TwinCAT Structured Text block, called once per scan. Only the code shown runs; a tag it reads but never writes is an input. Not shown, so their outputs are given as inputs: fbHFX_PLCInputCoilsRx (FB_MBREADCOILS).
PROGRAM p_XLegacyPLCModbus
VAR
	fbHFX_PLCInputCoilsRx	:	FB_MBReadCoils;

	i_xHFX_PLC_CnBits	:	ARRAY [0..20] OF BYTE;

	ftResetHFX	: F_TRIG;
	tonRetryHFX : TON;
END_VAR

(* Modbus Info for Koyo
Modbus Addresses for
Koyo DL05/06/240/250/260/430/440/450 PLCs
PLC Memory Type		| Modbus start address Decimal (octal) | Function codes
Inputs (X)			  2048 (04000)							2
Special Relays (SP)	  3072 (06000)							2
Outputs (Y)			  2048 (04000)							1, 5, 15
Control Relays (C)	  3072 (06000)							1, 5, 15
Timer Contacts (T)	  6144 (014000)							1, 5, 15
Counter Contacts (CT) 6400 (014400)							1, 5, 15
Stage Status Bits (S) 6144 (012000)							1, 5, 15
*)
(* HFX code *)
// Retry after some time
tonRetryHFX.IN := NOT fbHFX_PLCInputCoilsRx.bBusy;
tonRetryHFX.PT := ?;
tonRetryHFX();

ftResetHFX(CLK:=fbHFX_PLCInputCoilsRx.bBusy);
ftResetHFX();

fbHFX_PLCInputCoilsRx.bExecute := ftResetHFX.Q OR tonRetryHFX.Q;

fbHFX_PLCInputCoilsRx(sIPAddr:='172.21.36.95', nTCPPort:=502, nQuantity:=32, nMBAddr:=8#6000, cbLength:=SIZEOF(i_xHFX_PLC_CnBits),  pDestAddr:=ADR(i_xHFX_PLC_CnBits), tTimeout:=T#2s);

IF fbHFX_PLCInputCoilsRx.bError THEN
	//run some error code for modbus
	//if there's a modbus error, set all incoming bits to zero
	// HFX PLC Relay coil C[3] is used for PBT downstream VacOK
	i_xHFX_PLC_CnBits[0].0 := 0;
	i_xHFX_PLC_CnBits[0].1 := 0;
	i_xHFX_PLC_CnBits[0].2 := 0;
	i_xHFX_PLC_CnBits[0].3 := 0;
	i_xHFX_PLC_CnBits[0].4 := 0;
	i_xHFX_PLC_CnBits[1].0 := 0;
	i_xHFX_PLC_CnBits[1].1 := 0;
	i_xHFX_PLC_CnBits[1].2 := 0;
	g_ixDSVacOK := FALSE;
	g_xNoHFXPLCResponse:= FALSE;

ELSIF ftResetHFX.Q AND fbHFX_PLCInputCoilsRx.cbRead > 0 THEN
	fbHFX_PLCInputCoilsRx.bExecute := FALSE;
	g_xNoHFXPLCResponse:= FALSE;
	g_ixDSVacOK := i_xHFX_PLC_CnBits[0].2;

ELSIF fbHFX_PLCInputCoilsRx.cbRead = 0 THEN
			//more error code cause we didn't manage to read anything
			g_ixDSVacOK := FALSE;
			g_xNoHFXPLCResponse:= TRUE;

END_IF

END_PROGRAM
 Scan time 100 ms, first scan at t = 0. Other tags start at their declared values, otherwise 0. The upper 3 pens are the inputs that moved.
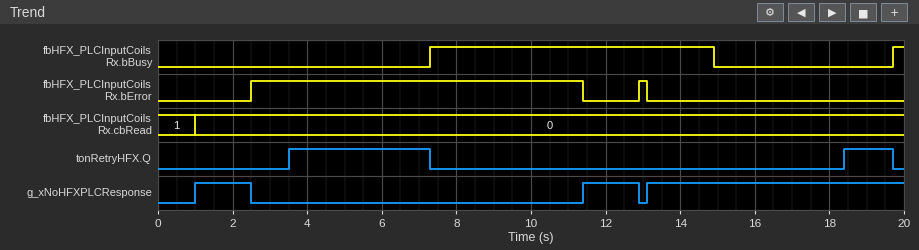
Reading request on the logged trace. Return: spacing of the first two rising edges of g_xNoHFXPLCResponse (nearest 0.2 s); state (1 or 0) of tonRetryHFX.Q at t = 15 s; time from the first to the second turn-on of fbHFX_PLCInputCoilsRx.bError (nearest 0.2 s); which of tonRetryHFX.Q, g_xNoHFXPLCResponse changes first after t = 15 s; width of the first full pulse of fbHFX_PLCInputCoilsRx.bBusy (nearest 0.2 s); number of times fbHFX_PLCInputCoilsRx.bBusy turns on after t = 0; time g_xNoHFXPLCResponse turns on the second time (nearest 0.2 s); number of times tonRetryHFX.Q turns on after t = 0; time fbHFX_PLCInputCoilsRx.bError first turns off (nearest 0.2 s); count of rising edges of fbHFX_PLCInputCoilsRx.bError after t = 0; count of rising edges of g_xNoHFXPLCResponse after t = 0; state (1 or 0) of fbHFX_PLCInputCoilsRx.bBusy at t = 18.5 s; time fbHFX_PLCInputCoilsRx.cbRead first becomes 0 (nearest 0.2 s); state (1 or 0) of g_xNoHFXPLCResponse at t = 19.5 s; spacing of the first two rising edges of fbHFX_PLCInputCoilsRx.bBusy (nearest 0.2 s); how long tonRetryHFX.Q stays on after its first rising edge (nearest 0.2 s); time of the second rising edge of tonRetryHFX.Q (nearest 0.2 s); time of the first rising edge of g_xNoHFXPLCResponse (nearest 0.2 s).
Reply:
10.4 s
0
10.4 s
tonRetryHFX.Q
7.6 s
2
11.4 s
2
11.4 s
2
3
0
1.0 s
1
12.4 s
3.8 s
18.4 s
1.0 s
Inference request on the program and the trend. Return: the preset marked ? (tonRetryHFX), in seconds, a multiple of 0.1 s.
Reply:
3.5 s
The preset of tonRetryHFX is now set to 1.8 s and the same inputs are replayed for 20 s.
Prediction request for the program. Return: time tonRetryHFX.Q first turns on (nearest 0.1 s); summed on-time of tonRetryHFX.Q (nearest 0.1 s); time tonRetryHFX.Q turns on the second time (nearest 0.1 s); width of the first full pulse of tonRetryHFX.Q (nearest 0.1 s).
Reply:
1.8 s
8.5 s
16.7 s
5.5 s
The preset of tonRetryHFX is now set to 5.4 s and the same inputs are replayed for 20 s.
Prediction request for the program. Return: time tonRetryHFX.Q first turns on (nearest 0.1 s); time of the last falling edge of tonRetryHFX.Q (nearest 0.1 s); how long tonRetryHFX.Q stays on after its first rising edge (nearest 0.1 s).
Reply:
5.4 s
7.3 s
1.9 s
